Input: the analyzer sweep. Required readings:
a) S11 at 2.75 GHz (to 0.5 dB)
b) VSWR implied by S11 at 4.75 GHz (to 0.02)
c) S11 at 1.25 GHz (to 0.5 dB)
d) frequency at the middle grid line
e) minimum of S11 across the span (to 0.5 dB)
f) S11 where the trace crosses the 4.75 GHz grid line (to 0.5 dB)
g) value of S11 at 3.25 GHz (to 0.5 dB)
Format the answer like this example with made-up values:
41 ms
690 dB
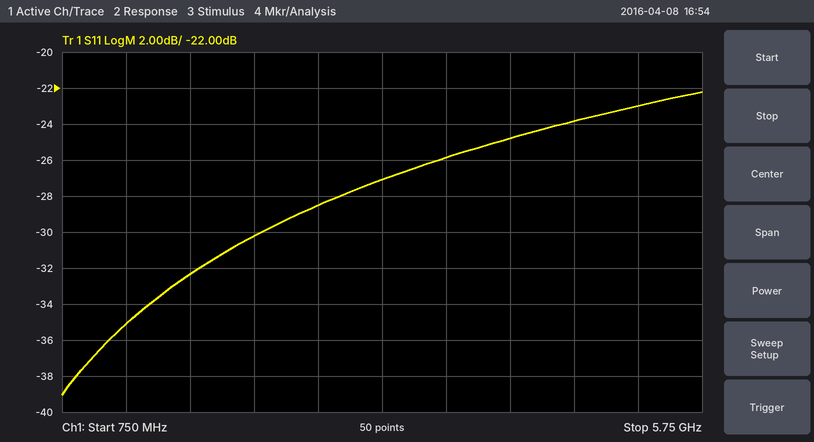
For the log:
-28.5 dB
1.14
-35.0 dB
3.25 GHz
-39.0 dB
-24.0 dB
-27.0 dB
